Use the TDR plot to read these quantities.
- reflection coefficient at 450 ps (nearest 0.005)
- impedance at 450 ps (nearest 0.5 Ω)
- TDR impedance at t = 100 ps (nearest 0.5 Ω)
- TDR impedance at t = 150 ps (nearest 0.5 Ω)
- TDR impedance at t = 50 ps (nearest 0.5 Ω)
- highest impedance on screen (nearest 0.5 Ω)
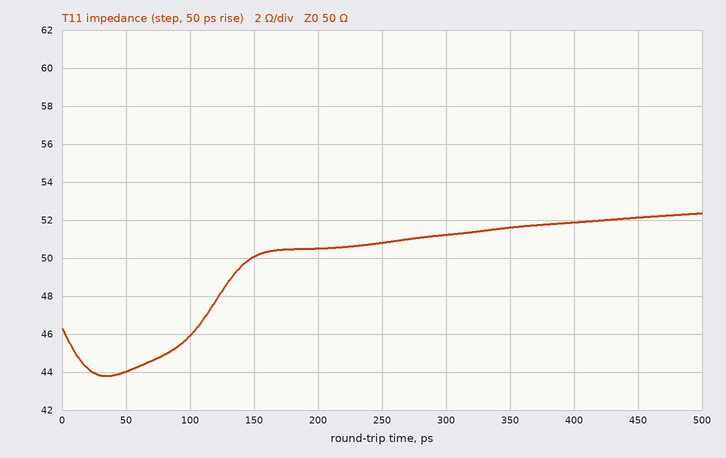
+0.020
52.0 Ω
46.0 Ω
50.0 Ω
44.0 Ω
52.5 Ω
